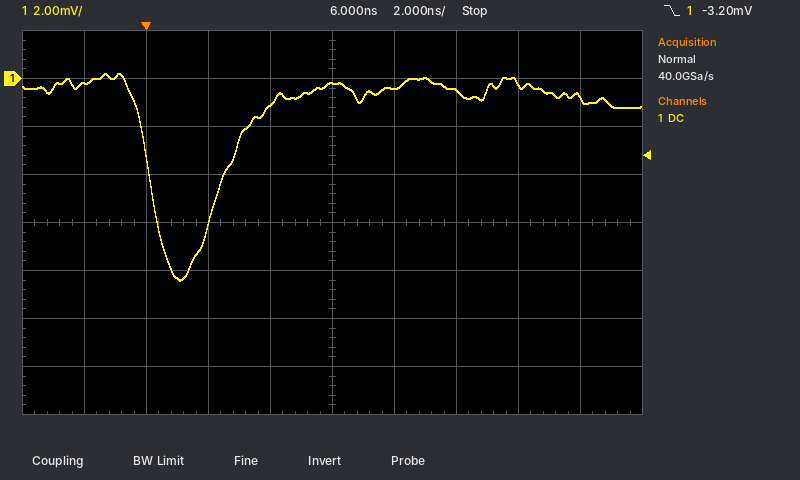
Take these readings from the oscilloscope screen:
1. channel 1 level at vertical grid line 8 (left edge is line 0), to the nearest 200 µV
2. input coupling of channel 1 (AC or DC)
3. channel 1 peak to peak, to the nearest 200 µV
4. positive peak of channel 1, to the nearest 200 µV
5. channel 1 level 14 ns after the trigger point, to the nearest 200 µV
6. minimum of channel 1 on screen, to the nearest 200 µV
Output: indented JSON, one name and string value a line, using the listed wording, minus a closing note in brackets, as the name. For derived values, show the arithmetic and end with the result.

{
  "channel 1 level at vertical grid line 8 (left edge is line 0), to the nearest 200 µV": "-200 µV",
  "input coupling of channel 1": "DC",
  "channel 1 peak to peak, to the nearest 200 µV": "200 µV − (-8.4 mV) = 8.6 mV",
  "positive peak of channel 1, to the nearest 200 µV": "200 µV",
  "channel 1 level 14 ns after the trigger point, to the nearest 200 µV": "-800 µV",
  "minimum of channel 1 on screen, to the nearest 200 µV": "-8.4 mV"
}
